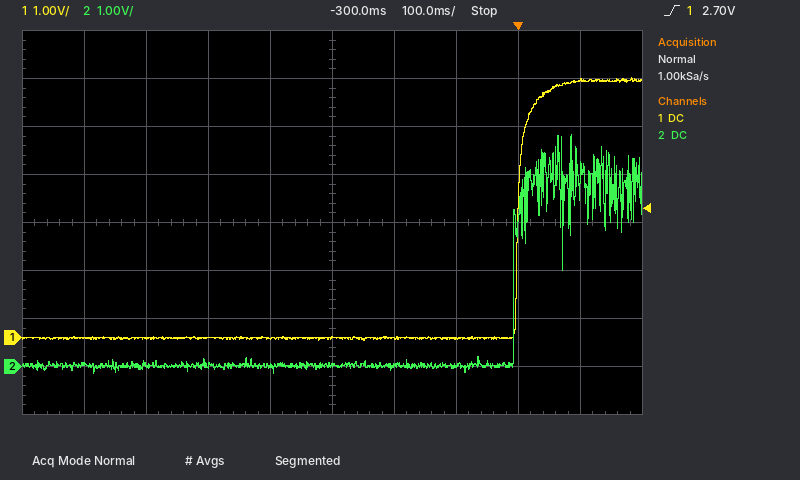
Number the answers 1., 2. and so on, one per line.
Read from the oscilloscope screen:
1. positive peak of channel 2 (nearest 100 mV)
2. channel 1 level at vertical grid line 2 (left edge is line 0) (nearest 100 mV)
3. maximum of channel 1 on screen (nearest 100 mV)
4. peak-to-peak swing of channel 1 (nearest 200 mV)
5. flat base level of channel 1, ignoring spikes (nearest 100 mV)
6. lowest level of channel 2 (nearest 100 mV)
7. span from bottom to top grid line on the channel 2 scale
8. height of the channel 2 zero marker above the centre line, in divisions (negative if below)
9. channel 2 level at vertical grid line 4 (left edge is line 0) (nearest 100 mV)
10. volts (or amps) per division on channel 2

1. 4.8 V
2. 0.0 V
3. 5.4 V
4. 5.4 V
5. 0.0 V
6. -100 mV
7. 8 V
8. -3.0 div
9. 0.0 V
10. 1 V
